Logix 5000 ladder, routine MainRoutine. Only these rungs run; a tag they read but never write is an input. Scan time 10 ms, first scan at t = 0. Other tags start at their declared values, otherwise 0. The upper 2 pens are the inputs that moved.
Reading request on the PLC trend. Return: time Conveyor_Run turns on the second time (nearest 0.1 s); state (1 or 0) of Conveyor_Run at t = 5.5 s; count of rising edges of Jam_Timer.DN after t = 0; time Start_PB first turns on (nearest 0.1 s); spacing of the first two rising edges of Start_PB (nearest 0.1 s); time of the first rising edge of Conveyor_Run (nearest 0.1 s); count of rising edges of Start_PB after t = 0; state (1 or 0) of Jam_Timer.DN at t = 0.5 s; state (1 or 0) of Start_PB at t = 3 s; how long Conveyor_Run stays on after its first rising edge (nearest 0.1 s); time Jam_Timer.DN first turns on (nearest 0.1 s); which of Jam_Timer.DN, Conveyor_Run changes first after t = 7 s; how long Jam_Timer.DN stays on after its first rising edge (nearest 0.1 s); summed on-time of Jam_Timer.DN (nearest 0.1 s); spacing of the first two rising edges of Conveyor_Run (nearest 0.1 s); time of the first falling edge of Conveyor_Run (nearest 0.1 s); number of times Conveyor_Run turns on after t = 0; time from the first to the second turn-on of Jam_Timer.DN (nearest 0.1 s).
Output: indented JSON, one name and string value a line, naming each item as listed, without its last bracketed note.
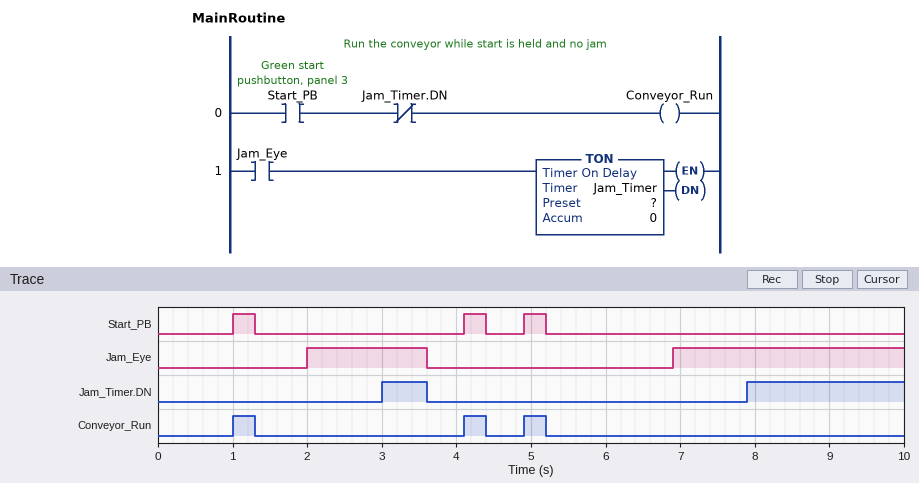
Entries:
{
  "time Conveyor_Run turns on the second time": "4.1 s",
  "state (1 or 0) of Conveyor_Run at t = 5.5 s": "0",
  "count of rising edges of Jam_Timer.DN after t = 0": "2",
  "time Start_PB first turns on": "1.0 s",
  "spacing of the first two rising edges of Start_PB": "3.1 s",
  "time of the first rising edge of Conveyor_Run": "1.0 s",
  "count of rising edges of Start_PB after t = 0": "3",
  "state (1 or 0) of Jam_Timer.DN at t = 0.5 s": "0",
  "state (1 or 0) of Start_PB at t = 3 s": "0",
  "how long Conveyor_Run stays on after its first rising edge": "0.3 s",
  "time Jam_Timer.DN first turns on": "3.0 s",
  "which of Jam_Timer.DN, Conveyor_Run changes first after t = 7 s": "Jam_Timer.DN",
  "how long Jam_Timer.DN stays on after its first rising edge": "0.6 s",
  "summed on-time of Jam_Timer.DN": "2.7 s",
  "spacing of the first two rising edges of Conveyor_Run": "3.1 s",
  "time of the first falling edge of Conveyor_Run": "1.3 s",
  "number of times Conveyor_Run turns on after t = 0": "3",
  "time from the first to the second turn-on of Jam_Timer.DN": "4.9 s"
}
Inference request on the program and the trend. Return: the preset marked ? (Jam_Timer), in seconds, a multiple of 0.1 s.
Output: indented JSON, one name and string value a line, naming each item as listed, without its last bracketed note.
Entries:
{
  "the preset marked ? (Jam_Timer), in seconds, a multiple of 0.1 s": "1.0 s"
}
